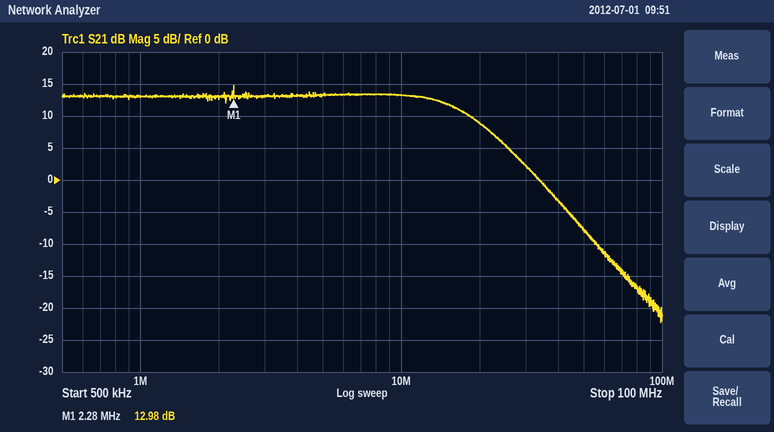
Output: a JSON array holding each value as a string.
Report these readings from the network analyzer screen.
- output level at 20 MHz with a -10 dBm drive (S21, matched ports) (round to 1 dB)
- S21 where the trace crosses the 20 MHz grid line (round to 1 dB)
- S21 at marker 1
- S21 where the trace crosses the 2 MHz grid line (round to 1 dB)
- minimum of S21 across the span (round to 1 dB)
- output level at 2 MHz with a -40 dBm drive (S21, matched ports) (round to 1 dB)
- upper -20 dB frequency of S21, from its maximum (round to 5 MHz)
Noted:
["-1 dBm", "9 dB", "12.98 dB", "13 dB", "-22 dB", "-27 dBm", "45 MHz"]
